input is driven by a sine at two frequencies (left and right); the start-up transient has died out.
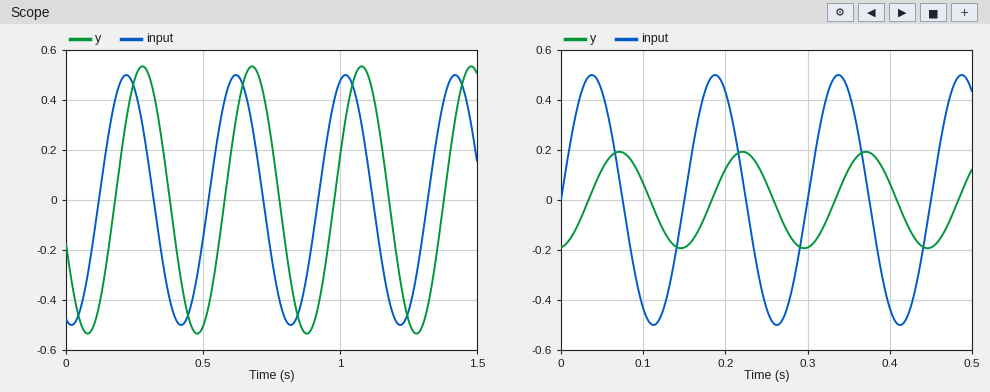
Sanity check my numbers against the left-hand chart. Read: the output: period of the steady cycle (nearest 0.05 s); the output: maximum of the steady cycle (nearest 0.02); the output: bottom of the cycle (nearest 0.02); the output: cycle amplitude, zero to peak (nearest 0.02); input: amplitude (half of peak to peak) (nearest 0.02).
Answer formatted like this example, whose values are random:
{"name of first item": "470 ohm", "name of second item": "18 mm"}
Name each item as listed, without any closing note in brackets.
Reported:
{"the output: period of the steady cycle": "0.40 s", "the output: maximum of the steady cycle": "0.54", "the output: bottom of the cycle": "-0.54", "the output: cycle amplitude, zero to peak": "0.54", "input: amplitude (half of peak to peak)": "0.50"}
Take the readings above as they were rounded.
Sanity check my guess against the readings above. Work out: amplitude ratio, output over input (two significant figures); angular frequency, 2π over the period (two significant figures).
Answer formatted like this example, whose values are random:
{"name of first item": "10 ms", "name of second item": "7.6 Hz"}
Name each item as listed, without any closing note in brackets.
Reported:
{"amplitude ratio, output over input": "1.1", "angular frequency, 2π over the period": "16 rad/s"}
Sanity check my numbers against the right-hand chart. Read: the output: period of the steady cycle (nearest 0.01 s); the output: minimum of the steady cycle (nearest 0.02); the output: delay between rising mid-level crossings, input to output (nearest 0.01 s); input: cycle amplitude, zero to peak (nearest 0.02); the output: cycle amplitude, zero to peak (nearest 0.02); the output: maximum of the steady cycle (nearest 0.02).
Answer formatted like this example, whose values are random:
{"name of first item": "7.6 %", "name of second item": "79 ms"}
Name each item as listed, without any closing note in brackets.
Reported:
{"the output: period of the steady cycle": "0.15 s", "the output: minimum of the steady cycle": "-0.20", "the output: delay between rising mid-level crossings, input to output": "0.03 s", "input: cycle amplitude, zero to peak": "0.50", "the output: cycle amplitude, zero to peak": "0.20", "the output: maximum of the steady cycle": "0.20"}
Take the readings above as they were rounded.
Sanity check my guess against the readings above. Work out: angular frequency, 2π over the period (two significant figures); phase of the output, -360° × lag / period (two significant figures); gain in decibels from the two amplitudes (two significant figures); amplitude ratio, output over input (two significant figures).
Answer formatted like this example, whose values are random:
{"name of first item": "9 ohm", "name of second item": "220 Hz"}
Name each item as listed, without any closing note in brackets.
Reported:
{"angular frequency, 2π over the period": "42 rad/s", "phase of the output, -360° × lag / period": "-72°", "gain in decibels from the two amplitudes": "-8.0 dB", "amplitude ratio, output over input": "0.40"}
